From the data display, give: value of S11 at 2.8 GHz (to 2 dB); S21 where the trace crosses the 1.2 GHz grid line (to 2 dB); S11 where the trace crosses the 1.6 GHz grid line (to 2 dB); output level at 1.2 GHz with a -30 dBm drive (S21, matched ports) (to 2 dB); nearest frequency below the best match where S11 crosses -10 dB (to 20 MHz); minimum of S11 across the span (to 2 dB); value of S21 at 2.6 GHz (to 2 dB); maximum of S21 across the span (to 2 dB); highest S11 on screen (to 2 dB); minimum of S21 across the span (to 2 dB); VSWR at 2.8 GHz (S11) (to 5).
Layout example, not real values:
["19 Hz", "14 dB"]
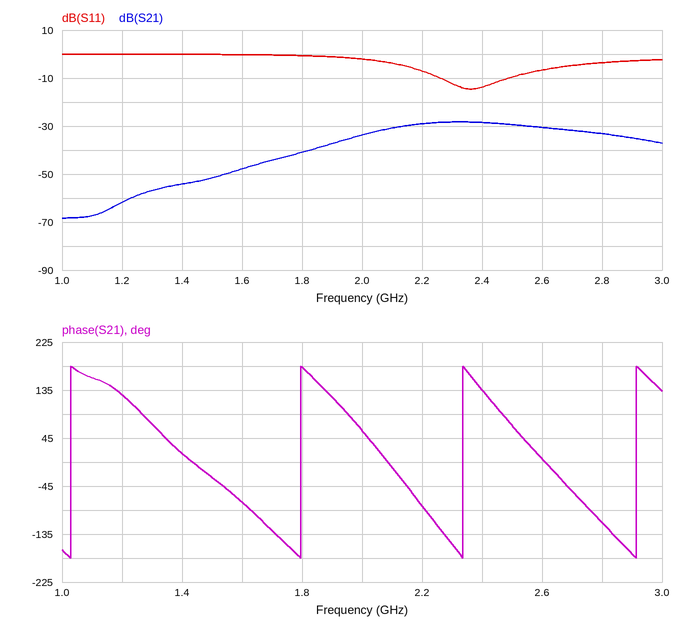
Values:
["-4 dB", "-62 dB", "0 dB", "-92 dBm", "2.26 GHz", "-14 dB", "-30 dB", "-28 dB", "0 dB", "-68 dB", "5"]
